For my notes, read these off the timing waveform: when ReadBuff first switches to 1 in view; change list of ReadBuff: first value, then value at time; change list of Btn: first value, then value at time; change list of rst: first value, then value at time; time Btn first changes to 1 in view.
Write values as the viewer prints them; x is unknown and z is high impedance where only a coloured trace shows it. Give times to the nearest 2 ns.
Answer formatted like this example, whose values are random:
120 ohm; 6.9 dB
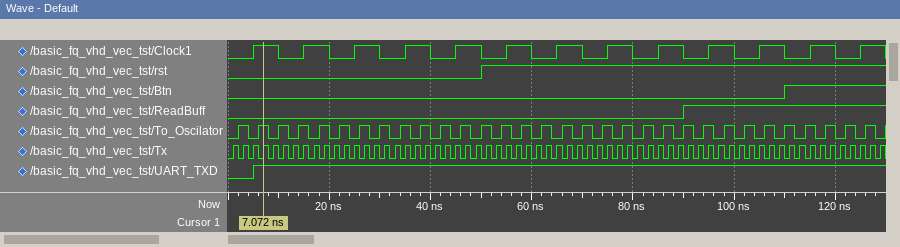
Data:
90 ns; 0, 1 at 90 ns; 0, 1 at 110 ns; 0, 1 at 50 ns; 110 ns
